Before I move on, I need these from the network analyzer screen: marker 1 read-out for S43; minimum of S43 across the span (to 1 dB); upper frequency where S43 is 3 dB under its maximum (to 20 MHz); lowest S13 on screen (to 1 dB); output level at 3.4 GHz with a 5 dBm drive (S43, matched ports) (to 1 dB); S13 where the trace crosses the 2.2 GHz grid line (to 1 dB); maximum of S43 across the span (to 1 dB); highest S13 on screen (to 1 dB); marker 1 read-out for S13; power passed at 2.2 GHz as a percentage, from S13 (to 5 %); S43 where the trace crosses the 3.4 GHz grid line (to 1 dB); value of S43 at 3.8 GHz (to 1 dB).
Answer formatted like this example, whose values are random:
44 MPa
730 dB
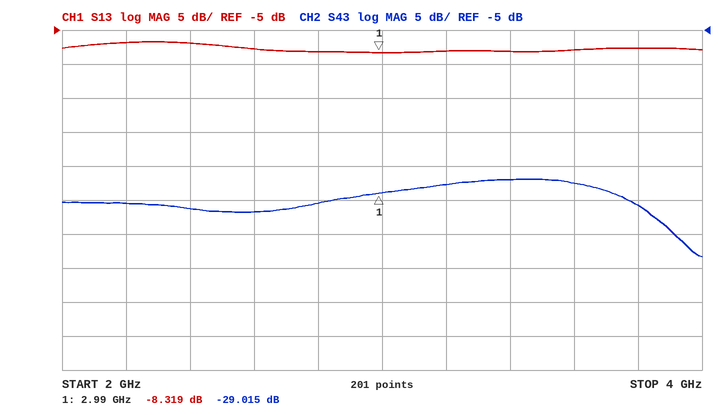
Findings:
-29.015 dB
-38 dB
3.76 GHz
-8 dB
-22 dBm
-7 dB
-27 dB
-7 dB
-8.319 dB
20 %
-27 dB
-31 dB
